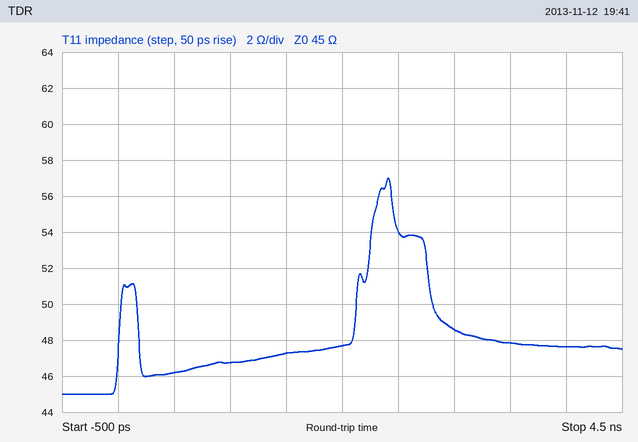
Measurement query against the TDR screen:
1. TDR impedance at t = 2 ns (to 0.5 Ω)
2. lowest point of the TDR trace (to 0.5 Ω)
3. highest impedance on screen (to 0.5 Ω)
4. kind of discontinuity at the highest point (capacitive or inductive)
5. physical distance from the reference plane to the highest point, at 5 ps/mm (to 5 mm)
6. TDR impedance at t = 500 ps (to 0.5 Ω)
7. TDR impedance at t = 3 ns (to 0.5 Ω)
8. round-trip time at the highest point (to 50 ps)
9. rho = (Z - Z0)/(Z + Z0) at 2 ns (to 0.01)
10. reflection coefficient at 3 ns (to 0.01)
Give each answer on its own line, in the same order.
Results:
47.5 Ω
45.0 Ω
57.0 Ω
inductive
240 mm
46.0 Ω
48.5 Ω
2.40 ns
+0.03
+0.04
